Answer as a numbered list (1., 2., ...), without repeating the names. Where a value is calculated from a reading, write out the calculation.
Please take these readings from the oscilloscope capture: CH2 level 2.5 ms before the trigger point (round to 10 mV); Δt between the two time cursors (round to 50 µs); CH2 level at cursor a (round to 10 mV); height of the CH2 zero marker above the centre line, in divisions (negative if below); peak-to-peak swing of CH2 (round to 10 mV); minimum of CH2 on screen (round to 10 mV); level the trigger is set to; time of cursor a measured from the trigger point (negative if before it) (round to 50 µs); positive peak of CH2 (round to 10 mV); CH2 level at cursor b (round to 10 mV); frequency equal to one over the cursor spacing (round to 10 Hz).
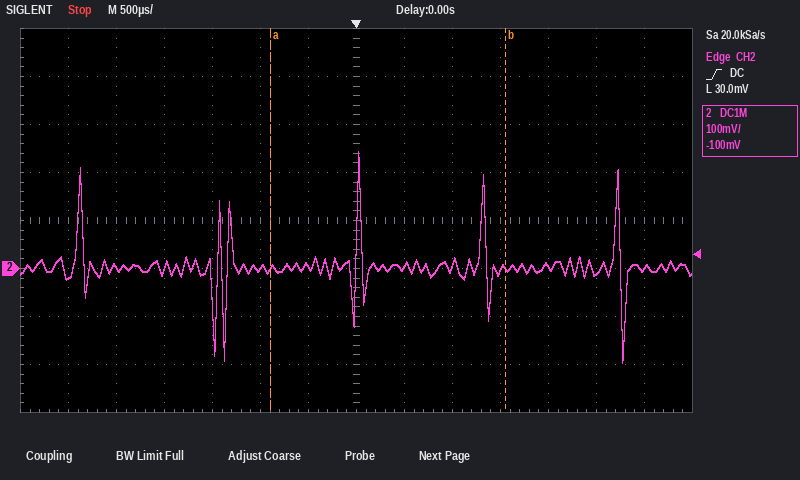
1. 0 mV
2. 2.45 ms
3. 0 mV
4. -1.0 div
5. 240 mV − (-200 mV) = 440 mV
6. -200 mV
7. 30.0 mV
8. -900 µs
9. 240 mV
10. 0 mV
11. 1 / 2.45 ms ≈ 410 Hz
